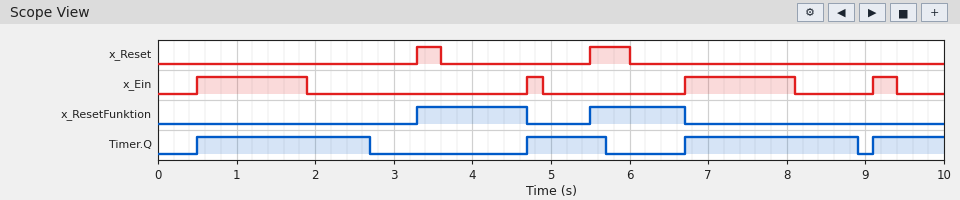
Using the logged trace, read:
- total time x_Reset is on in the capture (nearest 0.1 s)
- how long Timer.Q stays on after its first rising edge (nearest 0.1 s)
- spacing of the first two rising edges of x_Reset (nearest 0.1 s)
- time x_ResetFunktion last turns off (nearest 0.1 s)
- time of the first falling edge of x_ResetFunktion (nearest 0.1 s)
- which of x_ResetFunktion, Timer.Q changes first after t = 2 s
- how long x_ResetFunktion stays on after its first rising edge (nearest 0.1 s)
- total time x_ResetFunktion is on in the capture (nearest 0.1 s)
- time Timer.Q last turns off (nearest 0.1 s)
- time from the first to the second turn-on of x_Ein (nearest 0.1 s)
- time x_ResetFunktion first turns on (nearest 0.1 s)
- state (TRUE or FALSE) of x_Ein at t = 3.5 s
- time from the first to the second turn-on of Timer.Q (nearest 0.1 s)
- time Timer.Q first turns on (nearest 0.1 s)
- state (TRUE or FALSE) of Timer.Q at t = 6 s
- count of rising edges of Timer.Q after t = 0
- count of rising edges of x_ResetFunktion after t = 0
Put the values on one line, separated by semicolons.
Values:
0.8 s; 2.2 s; 2.2 s; 6.7 s; 4.7 s; Timer.Q; 1.4 s; 2.6 s; 8.9 s; 4.2 s; 3.3 s; FALSE; 4.2 s; 0.5 s; FALSE; 4; 2
